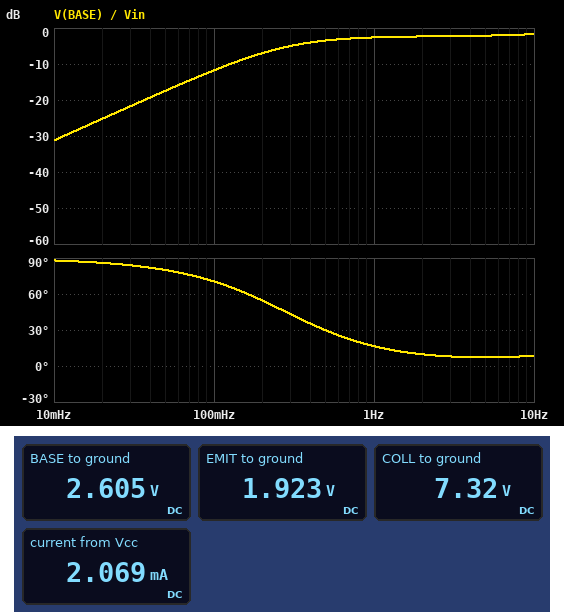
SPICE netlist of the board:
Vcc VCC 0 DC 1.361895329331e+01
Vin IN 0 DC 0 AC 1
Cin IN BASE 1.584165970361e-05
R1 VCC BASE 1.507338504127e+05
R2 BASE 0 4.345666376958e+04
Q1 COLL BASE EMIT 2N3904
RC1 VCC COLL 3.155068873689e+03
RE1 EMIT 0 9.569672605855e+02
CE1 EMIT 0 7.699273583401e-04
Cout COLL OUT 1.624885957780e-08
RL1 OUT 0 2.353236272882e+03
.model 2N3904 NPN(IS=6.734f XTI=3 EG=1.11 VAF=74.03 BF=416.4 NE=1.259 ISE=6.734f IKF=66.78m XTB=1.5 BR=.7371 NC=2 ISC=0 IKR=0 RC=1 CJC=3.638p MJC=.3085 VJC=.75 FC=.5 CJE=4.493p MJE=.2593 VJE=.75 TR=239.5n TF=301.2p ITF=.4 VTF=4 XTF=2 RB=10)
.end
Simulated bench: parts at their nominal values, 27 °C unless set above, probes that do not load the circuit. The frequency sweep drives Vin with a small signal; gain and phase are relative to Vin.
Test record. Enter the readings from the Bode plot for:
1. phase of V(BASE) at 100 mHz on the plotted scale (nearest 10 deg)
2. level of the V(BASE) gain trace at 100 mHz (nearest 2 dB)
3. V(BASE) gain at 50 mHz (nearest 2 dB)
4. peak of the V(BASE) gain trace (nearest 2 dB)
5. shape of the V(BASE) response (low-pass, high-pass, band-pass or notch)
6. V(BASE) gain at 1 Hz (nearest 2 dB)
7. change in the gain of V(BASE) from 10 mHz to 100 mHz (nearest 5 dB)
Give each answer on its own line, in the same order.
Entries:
70 deg
-12 dB
-18 dB
-2 dB
high-pass
-2 dB
20 dB
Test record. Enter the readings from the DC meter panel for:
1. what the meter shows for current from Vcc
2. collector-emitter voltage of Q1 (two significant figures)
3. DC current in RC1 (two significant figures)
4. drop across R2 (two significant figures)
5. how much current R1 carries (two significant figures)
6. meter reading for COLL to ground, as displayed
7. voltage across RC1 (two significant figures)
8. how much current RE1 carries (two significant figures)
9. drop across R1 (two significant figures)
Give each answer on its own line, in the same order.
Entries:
2.069 mA
5.4 V
2.0 mA
2.6 V
73 µA
7.32 V
6.3 V
2.0 mA
11 V
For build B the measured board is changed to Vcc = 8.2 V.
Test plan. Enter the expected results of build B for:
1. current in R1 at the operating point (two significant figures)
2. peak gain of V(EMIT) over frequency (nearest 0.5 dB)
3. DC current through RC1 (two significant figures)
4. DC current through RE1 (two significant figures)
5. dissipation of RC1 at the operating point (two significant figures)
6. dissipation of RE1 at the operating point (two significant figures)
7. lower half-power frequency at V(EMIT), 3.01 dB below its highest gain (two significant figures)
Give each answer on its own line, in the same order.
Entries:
44 µA
-3.0 dB
970 µA
980 µA
3.0 mW
910 µW
260 mHz
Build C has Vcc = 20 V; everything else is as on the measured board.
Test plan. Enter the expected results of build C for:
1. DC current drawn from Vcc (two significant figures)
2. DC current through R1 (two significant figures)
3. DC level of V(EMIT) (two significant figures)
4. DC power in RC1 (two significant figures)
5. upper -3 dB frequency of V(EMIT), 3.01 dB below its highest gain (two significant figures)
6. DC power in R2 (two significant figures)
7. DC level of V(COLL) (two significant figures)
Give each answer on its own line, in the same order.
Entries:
3.3 mA
110 µA
3.1 V
33 mW
29 Hz
330 µW
9.8 V
